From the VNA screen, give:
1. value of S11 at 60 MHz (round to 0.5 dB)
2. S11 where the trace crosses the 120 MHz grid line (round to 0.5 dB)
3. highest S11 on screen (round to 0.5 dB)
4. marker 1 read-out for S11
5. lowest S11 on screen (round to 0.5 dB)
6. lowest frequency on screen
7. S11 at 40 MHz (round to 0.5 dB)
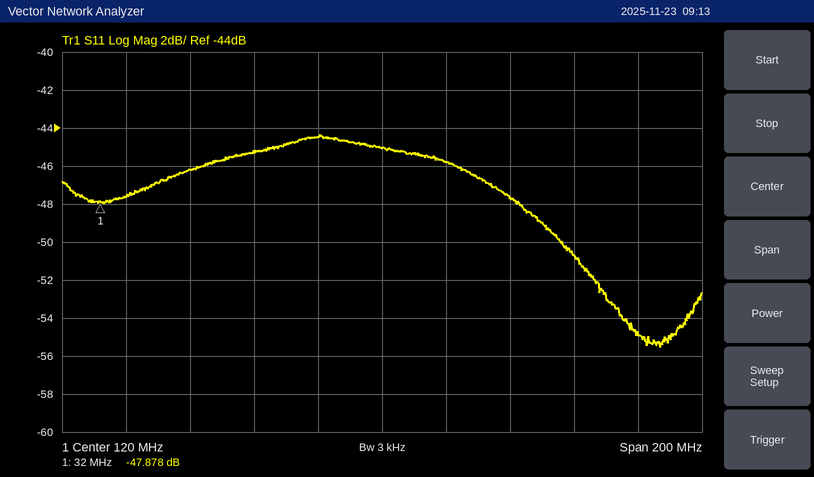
-46.0 dB
-45.0 dB
-44.5 dB
-47.878 dB
-55.5 dB
20 MHz
-47.5 dB
